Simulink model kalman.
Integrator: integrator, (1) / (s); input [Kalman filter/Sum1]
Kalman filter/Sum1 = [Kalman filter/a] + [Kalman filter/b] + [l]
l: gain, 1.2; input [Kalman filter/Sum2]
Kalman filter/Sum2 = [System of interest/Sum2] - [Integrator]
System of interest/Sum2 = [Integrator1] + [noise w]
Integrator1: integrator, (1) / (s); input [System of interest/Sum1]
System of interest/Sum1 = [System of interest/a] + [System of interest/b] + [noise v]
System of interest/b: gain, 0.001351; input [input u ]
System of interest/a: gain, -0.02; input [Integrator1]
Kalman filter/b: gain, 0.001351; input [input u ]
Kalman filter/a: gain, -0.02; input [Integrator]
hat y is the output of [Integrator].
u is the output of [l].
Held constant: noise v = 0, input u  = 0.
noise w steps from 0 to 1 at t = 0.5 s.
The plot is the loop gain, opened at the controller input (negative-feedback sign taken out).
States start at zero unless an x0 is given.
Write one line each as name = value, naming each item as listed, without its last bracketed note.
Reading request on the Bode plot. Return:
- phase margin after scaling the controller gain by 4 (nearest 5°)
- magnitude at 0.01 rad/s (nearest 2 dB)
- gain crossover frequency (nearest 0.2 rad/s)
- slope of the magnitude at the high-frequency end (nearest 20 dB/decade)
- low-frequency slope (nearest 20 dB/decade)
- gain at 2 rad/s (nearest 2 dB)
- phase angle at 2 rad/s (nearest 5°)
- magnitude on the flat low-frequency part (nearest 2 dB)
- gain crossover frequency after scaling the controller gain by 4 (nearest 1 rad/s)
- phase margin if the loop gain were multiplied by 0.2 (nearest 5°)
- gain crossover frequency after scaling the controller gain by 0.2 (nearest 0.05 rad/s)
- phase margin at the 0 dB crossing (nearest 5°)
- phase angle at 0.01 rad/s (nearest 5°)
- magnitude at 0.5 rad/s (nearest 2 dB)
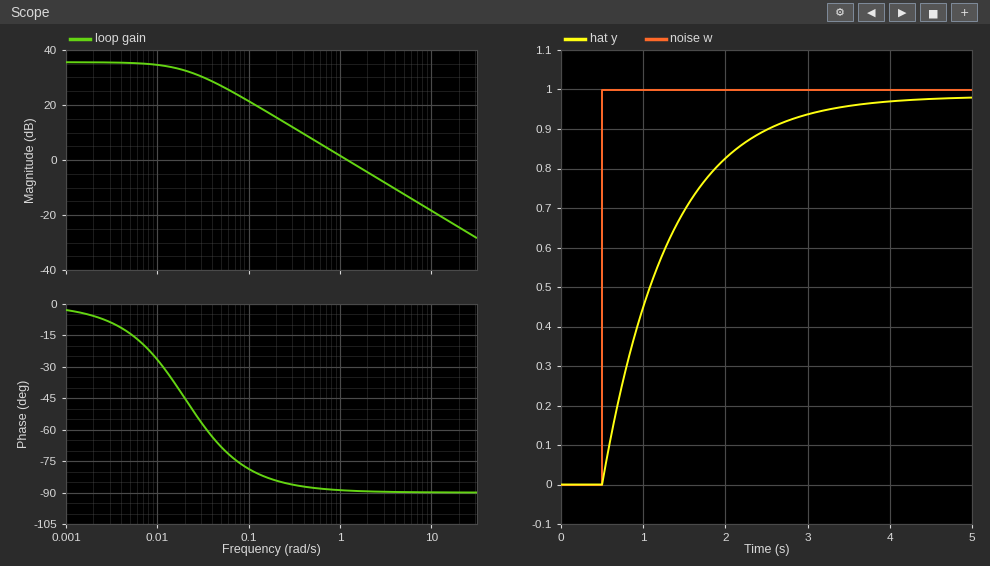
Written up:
phase margin after scaling the controller gain by 4 = 90°
magnitude at 0.01 rad/s = 34 dB
gain crossover frequency = 1.2 rad/s
slope of the magnitude at the high-frequency end = -20 dB/decade
low-frequency slope = 0 dB/decade
gain at 2 rad/s = -4 dB
phase angle at 2 rad/s = -90°
magnitude on the flat low-frequency part = 36 dB
gain crossover frequency after scaling the controller gain by 4 = 5 rad/s
phase margin if the loop gain were multiplied by 0.2 = 95°
gain crossover frequency after scaling the controller gain by 0.2 = 0.25 rad/s
phase margin at the 0 dB crossing = 90°
phase angle at 0.01 rad/s = -25°
magnitude at 0.5 rad/s = 8 dB
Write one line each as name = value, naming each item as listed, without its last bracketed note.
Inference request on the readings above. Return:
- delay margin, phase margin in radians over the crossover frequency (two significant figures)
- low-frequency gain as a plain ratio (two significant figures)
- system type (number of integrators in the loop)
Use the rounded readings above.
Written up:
delay margin, phase margin in radians over the crossover frequency = 1.3 s
low-frequency gain as a plain ratio = 63
system type = 0
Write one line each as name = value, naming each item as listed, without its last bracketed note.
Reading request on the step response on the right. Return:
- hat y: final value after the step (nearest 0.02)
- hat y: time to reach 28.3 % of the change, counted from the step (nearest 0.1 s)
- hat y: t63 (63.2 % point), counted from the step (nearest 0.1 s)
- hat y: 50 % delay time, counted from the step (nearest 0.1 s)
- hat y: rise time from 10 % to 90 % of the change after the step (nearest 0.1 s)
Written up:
hat y: final value after the step = 0.98
hat y: time to reach 28.3 % of the change, counted from the step = 0.3 s
hat y: t63 (63.2 % point), counted from the step = 0.8 s
hat y: 50 % delay time, counted from the step = 0.6 s
hat y: rise time from 10 % to 90 % of the change after the step = 1.8 s
